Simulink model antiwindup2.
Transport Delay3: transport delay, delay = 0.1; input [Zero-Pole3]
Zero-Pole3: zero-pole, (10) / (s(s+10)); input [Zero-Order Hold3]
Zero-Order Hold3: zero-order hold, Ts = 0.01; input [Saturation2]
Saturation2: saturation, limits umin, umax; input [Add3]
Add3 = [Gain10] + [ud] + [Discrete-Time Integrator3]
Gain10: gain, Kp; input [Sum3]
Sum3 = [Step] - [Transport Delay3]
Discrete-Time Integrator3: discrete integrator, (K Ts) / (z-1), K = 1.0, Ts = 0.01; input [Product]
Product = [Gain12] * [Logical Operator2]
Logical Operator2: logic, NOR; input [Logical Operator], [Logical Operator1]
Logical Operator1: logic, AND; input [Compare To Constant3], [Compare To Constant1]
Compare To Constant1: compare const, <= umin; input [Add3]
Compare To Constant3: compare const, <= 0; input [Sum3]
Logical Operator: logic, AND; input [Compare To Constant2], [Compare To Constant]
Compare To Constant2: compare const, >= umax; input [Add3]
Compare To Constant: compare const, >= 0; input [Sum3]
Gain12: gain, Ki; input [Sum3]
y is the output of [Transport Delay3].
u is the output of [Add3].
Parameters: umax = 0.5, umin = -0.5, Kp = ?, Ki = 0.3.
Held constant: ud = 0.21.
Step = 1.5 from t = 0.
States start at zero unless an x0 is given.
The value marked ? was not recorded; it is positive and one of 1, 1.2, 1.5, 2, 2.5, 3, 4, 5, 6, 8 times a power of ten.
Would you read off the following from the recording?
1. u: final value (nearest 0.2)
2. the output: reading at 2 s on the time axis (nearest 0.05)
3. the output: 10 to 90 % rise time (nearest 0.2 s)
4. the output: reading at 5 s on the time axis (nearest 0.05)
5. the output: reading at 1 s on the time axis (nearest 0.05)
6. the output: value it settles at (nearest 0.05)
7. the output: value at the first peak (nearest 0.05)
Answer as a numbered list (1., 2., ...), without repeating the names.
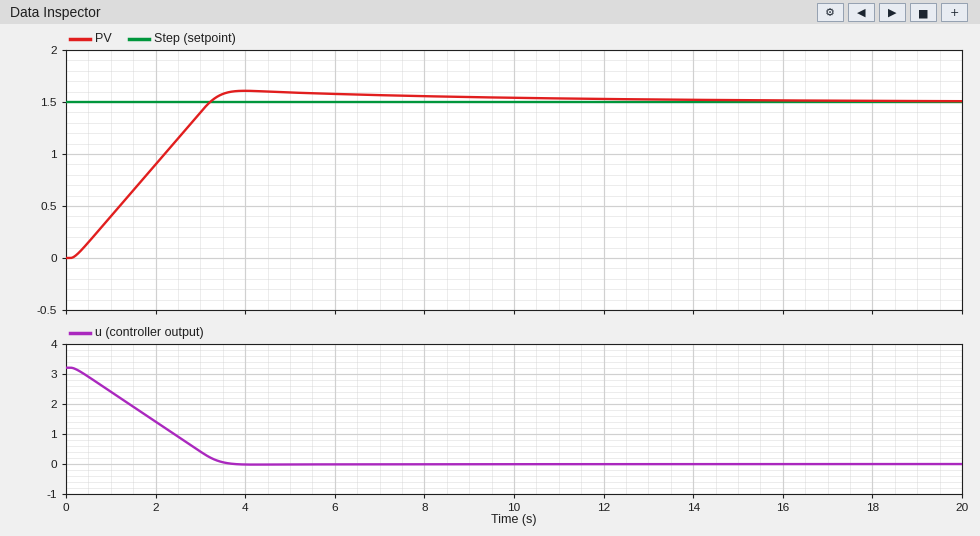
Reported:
1. 0.0
2. 0.90
3. 2.4 s
4. 1.60
5. 0.40
6. 1.50
7. 1.60
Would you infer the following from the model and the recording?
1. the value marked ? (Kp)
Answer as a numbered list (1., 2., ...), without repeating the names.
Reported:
1. 2
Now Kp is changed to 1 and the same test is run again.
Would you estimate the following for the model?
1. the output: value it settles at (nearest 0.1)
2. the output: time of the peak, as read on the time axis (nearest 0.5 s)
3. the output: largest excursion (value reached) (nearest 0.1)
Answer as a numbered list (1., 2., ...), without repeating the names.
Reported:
1. 1.5
2. 5.0 s
3. 1.7
